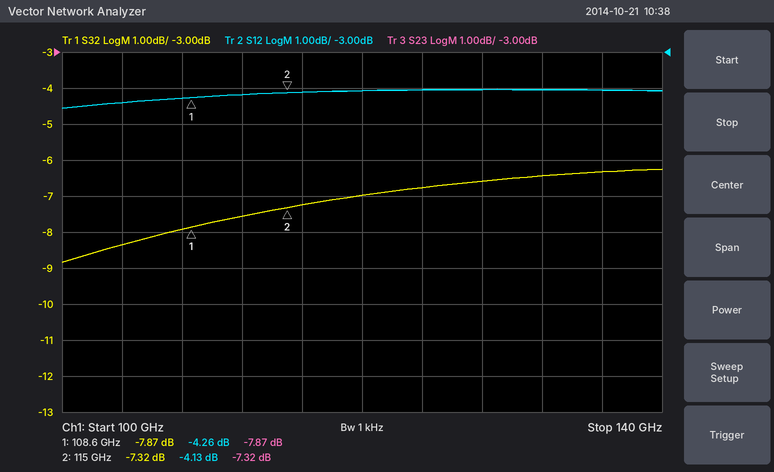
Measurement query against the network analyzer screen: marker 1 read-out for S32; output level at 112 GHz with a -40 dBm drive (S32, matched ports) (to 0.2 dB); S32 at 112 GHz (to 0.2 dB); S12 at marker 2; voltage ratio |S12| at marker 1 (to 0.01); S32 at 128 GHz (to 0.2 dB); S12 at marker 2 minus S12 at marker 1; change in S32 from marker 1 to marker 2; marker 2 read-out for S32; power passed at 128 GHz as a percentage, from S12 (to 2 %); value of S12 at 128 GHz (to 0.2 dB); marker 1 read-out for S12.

-7.87 dB
-47.6 dBm
-7.6 dB
-4.13 dB
0.61
-6.6 dB
0.13 dB
0.55 dB
-7.32 dB
40 %
-4.0 dB
-4.26 dB
